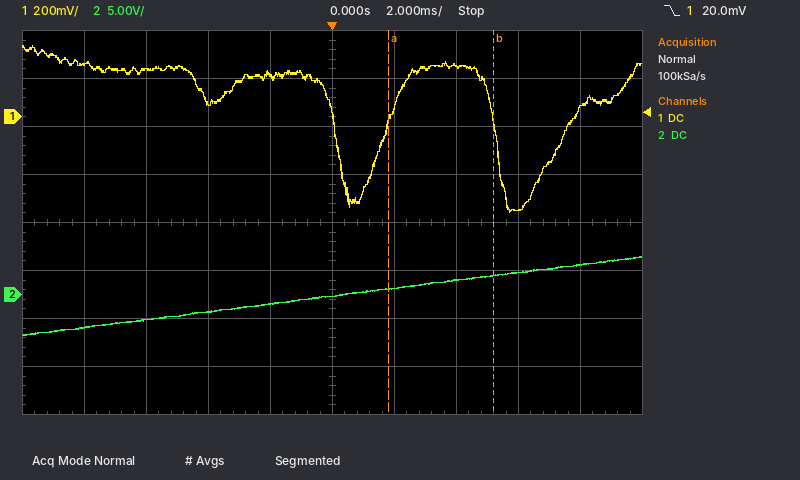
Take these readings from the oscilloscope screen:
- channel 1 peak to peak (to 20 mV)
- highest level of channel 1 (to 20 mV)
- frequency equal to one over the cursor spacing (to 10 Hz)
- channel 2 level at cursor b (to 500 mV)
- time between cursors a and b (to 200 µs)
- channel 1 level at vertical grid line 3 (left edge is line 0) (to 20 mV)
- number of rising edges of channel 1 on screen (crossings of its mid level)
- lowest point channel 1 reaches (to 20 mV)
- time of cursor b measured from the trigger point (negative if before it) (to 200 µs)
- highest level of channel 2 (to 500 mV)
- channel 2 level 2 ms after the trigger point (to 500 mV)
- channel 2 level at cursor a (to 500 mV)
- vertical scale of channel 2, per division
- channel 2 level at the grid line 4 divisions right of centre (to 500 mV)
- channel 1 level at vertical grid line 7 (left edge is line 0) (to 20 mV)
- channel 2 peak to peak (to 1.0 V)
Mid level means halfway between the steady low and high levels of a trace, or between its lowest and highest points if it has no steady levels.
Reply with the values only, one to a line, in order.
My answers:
700 mV
300 mV
290 Hz
2.0 V
3.4 ms
60 mV
2
-400 mV
+5.2 ms
4.0 V
500 mV
500 mV
5 V
3.0 V
220 mV
8.0 V
